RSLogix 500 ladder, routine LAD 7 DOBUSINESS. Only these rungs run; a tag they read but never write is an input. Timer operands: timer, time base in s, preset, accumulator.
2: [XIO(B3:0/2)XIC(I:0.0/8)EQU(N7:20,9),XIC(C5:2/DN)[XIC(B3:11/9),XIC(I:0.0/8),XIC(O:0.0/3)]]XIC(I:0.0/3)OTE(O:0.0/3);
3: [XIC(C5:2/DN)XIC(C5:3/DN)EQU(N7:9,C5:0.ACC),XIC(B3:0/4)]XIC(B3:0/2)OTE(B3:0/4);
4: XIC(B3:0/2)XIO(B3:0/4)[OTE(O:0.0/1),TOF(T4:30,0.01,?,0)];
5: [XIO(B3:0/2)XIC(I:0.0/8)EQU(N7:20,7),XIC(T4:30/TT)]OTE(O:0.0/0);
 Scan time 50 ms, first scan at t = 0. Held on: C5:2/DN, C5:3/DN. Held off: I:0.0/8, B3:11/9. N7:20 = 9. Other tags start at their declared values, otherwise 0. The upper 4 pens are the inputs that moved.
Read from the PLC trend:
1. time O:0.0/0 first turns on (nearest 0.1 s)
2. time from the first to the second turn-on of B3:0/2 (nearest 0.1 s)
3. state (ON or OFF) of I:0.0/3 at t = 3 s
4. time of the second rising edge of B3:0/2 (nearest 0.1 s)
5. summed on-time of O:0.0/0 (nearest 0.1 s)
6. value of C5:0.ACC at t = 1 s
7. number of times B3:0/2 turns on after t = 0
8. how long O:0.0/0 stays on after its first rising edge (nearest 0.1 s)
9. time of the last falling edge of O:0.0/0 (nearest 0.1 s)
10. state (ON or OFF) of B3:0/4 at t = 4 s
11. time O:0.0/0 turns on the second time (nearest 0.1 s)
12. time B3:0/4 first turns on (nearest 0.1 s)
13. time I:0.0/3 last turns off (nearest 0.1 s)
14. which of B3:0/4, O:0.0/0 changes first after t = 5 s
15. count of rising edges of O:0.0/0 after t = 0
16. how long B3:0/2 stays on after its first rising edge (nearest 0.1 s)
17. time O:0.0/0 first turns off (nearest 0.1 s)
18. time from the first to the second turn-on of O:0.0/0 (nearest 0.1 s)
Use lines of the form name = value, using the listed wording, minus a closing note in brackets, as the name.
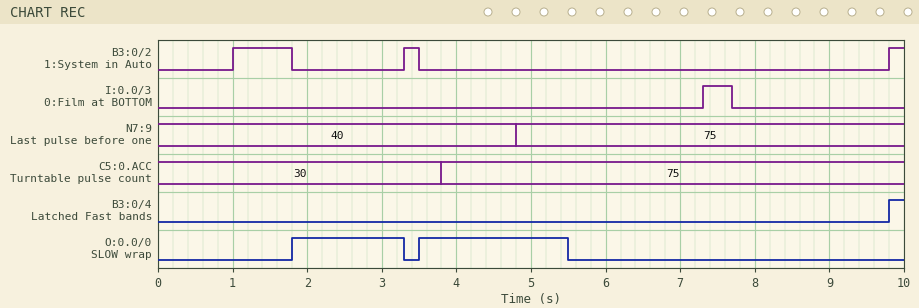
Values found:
time O:0.0/0 first turns on = 1.8 s
time from the first to the second turn-on of B3:0/2 = 2.3 s
state (ON or OFF) of I:0.0/3 at t = 3 s = OFF
time of the second rising edge of B3:0/2 = 3.3 s
summed on-time of O:0.0/0 = 3.5 s
value of C5:0.ACC at t = 1 s = 30
number of times B3:0/2 turns on after t = 0 = 3
how long O:0.0/0 stays on after its first rising edge = 1.5 s
time of the last falling edge of O:0.0/0 = 5.5 s
state (ON or OFF) of B3:0/4 at t = 4 s = OFF
time O:0.0/0 turns on the second time = 3.5 s
time B3:0/4 first turns on = 9.8 s
time I:0.0/3 last turns off = 7.7 s
which of B3:0/4, O:0.0/0 changes first after t = 5 s = O:0.0/0
count of rising edges of O:0.0/0 after t = 0 = 2
how long B3:0/2 stays on after its first rising edge = 0.8 s
time O:0.0/0 first turns off = 3.3 s
time from the first to the second turn-on of O:0.0/0 = 1.7 s
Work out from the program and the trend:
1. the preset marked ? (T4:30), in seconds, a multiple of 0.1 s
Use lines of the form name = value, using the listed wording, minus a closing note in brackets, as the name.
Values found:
the preset marked ? (T4:30), in seconds, a multiple of 0.1 s = 2.0 s
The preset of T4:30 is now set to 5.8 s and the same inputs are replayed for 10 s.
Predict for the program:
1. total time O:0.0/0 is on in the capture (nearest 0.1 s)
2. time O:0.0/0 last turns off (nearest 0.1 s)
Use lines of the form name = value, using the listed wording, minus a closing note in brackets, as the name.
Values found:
total time O:0.0/0 is on in the capture = 7.3 s
time O:0.0/0 last turns off = 9.3 s
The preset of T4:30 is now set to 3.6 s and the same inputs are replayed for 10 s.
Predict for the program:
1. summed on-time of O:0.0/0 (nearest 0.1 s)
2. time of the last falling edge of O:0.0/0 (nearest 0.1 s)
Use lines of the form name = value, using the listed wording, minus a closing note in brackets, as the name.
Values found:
summed on-time of O:0.0/0 = 5.1 s
time of the last falling edge of O:0.0/0 = 7.1 s
